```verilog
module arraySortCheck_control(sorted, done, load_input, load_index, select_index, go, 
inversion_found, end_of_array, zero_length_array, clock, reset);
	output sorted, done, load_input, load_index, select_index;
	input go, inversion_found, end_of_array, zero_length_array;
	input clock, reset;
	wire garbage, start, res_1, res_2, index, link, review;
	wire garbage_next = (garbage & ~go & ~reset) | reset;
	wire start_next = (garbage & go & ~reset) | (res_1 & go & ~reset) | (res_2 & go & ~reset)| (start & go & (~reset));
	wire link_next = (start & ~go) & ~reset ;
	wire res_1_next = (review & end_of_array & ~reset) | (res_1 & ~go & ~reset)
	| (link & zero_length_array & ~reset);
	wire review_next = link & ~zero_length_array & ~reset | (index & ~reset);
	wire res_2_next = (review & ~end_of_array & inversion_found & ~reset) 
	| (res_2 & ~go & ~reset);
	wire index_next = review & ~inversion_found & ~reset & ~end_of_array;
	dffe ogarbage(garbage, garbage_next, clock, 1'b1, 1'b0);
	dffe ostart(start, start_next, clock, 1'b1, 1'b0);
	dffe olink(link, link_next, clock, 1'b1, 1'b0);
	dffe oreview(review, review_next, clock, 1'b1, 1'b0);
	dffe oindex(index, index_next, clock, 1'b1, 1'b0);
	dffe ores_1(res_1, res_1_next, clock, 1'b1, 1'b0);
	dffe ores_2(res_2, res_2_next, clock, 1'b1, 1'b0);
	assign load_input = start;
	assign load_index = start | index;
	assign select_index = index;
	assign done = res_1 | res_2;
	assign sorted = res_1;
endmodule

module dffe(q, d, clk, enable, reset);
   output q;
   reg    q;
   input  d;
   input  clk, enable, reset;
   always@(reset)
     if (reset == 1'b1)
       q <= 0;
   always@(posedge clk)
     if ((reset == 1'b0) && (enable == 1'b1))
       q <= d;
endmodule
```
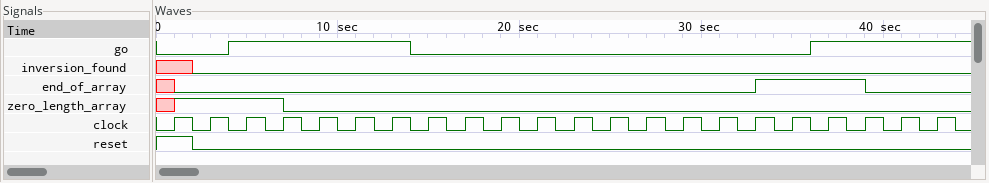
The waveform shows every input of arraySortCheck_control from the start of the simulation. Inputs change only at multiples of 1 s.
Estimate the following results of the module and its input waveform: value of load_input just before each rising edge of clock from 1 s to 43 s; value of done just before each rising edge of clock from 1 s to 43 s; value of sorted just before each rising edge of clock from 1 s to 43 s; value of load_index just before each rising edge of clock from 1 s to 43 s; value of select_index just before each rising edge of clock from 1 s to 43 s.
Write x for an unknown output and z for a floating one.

x 0 0 1 1 1 1 1 0 0 0 0 0 0 0 0 0 0 0 1 1 1
x 0 0 0 0 0 0 0 0 0 0 0 0 0 0 0 0 0 1 0 0 0
x 0 0 0 0 0 0 0 0 0 0 0 0 0 0 0 0 0 1 0 0 0
x 0 0 1 1 1 1 1 0 0 1 0 1 0 1 0 1 0 0 1 1 1
x 0 0 0 0 0 0 0 0 0 1 0 1 0 1 0 1 0 0 0 0 0
